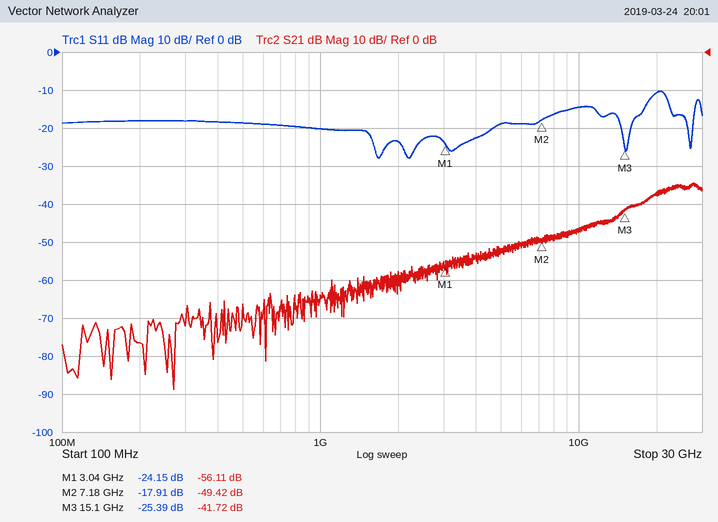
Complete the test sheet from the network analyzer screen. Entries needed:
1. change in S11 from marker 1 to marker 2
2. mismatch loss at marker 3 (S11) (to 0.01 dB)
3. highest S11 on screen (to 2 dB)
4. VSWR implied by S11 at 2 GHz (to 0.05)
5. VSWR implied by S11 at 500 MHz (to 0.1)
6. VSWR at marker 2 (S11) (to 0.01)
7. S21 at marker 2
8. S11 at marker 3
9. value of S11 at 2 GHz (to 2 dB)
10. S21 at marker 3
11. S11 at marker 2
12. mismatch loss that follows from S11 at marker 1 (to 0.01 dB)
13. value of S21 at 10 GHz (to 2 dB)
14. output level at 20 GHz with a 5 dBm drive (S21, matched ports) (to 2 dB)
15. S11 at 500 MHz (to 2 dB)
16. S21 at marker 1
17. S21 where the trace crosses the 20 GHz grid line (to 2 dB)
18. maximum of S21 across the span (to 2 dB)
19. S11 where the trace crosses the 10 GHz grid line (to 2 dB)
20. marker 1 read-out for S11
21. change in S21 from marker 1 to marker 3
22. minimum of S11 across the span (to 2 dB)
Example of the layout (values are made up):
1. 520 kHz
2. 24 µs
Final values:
1. 6.24 dB
2. 0.01 dB
3. -10 dB
4. 1.15
5. 1.3
6. 1.29
7. -49.42 dB
8. -25.39 dB
9. -24 dB
10. -41.72 dB
11. -17.91 dB
12. 0.02 dB
13. -46 dB
14. -32 dBm
15. -18 dB
16. -56.11 dB
17. -38 dB
18. -34 dB
19. -14 dB
20. -24.15 dB
21. 14.39 dB
22. -28 dB
